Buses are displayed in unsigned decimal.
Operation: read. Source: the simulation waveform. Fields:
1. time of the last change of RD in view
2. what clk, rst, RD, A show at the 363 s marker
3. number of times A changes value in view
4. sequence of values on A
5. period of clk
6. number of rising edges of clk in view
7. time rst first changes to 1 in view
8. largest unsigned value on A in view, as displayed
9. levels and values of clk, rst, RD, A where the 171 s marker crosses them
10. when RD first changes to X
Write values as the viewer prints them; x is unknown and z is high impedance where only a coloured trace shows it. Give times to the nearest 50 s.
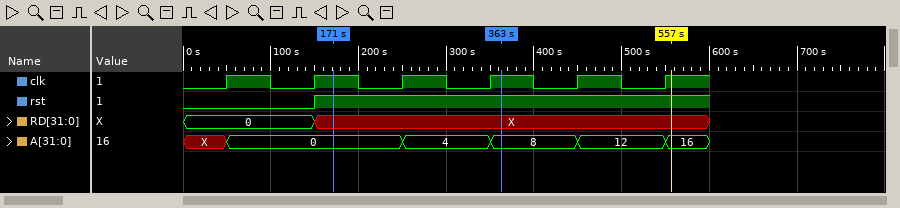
150 s
clk=1, rst=1, RD=X, A=8
5
X, 0, 4, 8, 12, 16
100 s
6
150 s
16
clk=1, rst=1, RD=X, A=0
150 s
